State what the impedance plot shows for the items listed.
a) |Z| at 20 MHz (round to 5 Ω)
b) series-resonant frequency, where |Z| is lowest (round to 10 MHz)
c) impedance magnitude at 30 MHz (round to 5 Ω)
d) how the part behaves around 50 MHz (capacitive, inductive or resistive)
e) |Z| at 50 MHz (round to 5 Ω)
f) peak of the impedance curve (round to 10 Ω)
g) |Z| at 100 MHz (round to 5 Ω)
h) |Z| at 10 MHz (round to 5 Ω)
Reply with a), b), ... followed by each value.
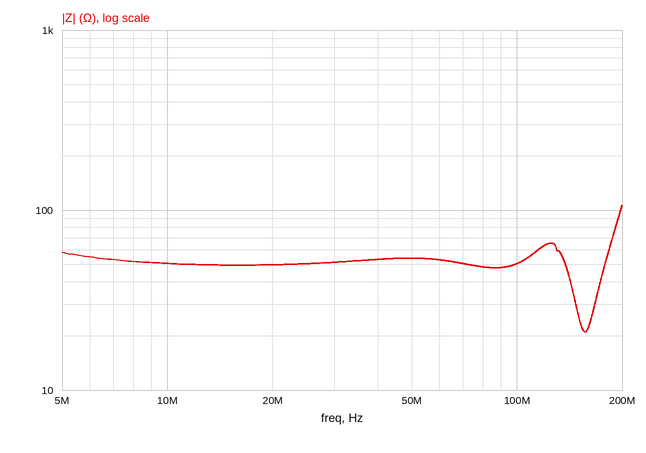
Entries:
a) 50 Ω
b) 160 MHz
c) 50 Ω
d) resistive
e) 55 Ω
f) 110 Ω
g) 50 Ω
h) 50 Ω
